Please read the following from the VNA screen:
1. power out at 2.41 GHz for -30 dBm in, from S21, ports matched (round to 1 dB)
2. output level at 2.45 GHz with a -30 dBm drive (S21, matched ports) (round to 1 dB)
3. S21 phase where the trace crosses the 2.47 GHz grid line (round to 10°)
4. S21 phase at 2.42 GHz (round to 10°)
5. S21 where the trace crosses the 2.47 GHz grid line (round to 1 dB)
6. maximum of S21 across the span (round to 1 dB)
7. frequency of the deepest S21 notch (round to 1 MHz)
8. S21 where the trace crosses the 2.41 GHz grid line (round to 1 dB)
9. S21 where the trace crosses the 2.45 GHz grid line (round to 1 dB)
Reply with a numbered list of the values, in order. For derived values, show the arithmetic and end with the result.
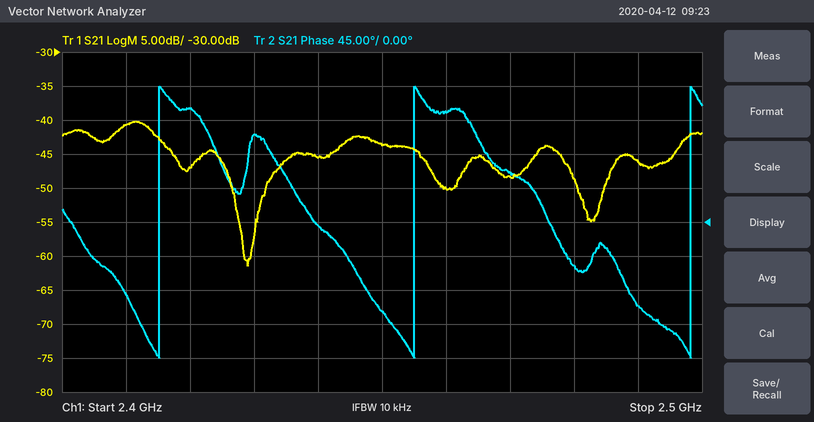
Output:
1. -30 dBm + (-41 dB) = -71 dBm
2. -30 dBm + (-44 dB) = -74 dBm
3. 70°
4. 150°
5. -48 dB
6. -40 dB
7. 2.429 GHz
8. -41 dB
9. -44 dB
